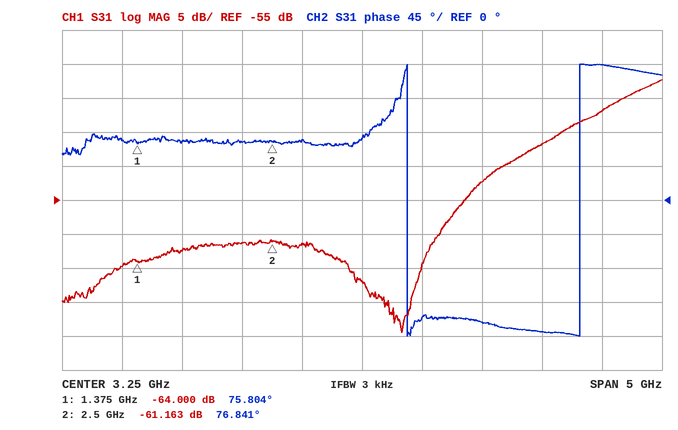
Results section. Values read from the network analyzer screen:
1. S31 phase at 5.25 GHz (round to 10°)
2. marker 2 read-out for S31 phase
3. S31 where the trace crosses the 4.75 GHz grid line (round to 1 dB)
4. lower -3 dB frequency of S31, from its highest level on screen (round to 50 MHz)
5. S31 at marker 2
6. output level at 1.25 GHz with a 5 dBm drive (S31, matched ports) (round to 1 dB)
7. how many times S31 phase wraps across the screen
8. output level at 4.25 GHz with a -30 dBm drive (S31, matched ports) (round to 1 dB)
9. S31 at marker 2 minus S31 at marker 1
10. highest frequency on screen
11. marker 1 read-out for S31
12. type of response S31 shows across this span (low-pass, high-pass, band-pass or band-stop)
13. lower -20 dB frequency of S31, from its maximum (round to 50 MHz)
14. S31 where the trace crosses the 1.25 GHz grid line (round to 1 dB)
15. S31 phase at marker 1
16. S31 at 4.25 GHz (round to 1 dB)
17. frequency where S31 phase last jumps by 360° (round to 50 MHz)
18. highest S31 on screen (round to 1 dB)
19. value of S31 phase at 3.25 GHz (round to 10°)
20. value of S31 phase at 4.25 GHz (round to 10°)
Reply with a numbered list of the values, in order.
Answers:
1. 180°
2. 76.841°
3. -47 dB
4. 5.40 GHz
5. -61.163 dB
6. -60 dBm
7. 2
8. -82 dBm
9. 2.837 dB
10. 5.75 GHz
11. -64.000 dB
12. high-pass
13. 4.00 GHz
14. -65 dB
15. 75.804°
16. -52 dB
17. 5.05 GHz
18. -37 dB
19. 80°
20. -160°
